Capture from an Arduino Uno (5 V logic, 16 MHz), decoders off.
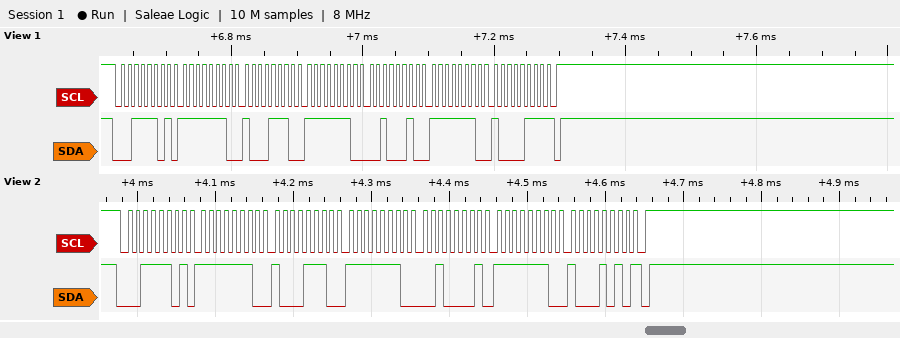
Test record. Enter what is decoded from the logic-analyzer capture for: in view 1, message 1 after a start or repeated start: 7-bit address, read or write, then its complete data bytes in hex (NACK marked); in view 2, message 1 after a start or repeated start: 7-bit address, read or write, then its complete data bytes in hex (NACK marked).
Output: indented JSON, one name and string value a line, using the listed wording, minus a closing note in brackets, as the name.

{
  "in view 1, message 1 after a start or repeated start: 7-bit address, read or write, then its complete data bytes in hex": "0x1E read: FE 8E FE 22 FE 87 NACK",
  "in view 2, message 1 after a start or repeated start: 7-bit address, read or write, then its complete data bytes in hex": "0x1E read: FE 8E FE 21 FE 8A NACK"
}
